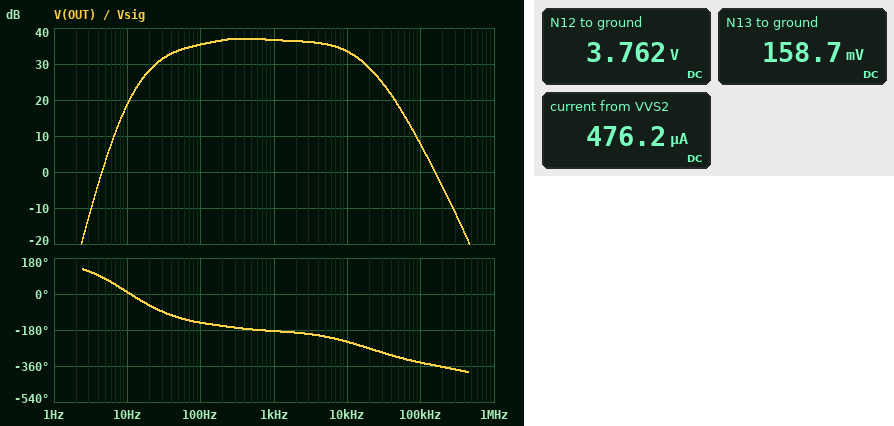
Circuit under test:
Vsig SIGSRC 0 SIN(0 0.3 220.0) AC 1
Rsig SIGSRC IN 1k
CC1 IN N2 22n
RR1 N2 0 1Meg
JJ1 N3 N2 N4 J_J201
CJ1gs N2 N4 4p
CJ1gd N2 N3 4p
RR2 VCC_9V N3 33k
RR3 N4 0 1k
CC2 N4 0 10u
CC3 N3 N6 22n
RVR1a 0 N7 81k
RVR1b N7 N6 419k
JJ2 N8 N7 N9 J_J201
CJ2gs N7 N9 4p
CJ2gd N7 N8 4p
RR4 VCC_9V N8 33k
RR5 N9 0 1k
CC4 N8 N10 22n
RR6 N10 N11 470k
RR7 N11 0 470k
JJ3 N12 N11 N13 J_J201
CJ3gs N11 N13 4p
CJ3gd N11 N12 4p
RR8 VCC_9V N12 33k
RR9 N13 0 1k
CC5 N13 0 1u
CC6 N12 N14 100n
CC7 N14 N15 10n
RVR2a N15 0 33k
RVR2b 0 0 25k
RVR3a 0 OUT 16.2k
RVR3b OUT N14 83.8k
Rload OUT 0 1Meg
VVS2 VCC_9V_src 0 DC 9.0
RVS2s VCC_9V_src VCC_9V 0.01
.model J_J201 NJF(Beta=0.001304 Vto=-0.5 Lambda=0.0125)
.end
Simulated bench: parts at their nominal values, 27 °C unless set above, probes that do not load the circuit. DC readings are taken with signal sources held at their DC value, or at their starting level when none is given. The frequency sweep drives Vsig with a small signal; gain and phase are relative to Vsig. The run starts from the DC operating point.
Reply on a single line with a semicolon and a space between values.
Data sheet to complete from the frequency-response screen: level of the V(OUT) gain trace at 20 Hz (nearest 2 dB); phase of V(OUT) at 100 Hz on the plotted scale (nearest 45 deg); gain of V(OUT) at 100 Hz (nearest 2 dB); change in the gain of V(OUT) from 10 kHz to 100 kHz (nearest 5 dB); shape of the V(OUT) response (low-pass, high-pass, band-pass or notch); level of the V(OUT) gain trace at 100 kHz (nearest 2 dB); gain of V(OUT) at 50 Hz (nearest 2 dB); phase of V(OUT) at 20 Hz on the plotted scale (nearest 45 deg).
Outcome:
28 dB; -135 deg; 36 dB; -25 dB; band-pass; 8 dB; 34 dB; -45 deg
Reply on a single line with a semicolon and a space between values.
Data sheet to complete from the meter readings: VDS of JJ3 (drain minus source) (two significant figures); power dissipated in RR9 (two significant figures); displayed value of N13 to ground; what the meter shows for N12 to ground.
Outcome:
3.6 V; 25 µW; 158.7 mV; 3.762 V
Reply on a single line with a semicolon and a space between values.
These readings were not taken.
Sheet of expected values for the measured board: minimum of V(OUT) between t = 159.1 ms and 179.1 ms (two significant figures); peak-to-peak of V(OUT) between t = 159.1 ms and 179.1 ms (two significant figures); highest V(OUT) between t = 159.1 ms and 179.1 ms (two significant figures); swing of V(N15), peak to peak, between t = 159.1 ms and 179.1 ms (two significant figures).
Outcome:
-660 mV; 1.2 V; 550 mV; 11 V
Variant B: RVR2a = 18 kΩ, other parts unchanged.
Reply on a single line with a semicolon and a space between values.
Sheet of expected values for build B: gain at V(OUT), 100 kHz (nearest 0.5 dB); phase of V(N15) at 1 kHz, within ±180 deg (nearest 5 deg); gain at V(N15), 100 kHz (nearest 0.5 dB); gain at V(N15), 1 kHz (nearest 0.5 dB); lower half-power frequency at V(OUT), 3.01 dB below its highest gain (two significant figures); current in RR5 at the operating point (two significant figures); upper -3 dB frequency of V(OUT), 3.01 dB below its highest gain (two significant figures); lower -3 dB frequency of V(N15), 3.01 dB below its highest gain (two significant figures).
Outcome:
7.0 dB; -155 deg; 23.0 dB; 48.5 dB; 57 Hz; 160 µA; 1.9 kHz; 470 Hz
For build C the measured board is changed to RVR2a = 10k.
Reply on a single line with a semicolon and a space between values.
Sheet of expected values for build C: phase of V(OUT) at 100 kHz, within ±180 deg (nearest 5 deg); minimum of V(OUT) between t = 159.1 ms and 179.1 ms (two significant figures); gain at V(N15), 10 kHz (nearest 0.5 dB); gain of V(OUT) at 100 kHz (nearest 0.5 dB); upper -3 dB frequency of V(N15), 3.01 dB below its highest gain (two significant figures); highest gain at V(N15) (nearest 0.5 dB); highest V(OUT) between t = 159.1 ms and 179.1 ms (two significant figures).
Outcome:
20 deg; -620 mV; 45.0 dB; 6.5 dB; 17 kHz; 46.0 dB; 570 mV
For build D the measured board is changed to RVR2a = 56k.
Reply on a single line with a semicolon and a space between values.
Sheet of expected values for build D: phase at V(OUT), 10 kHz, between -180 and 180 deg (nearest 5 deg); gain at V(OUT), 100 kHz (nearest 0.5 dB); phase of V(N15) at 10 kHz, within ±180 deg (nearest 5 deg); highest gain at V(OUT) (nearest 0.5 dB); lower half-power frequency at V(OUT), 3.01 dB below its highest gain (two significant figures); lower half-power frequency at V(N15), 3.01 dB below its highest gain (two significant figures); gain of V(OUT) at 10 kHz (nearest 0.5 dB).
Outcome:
115 deg; 8.0 dB; 120 deg; 38.0 dB; 84 Hz; 330 Hz; 34.5 dB
